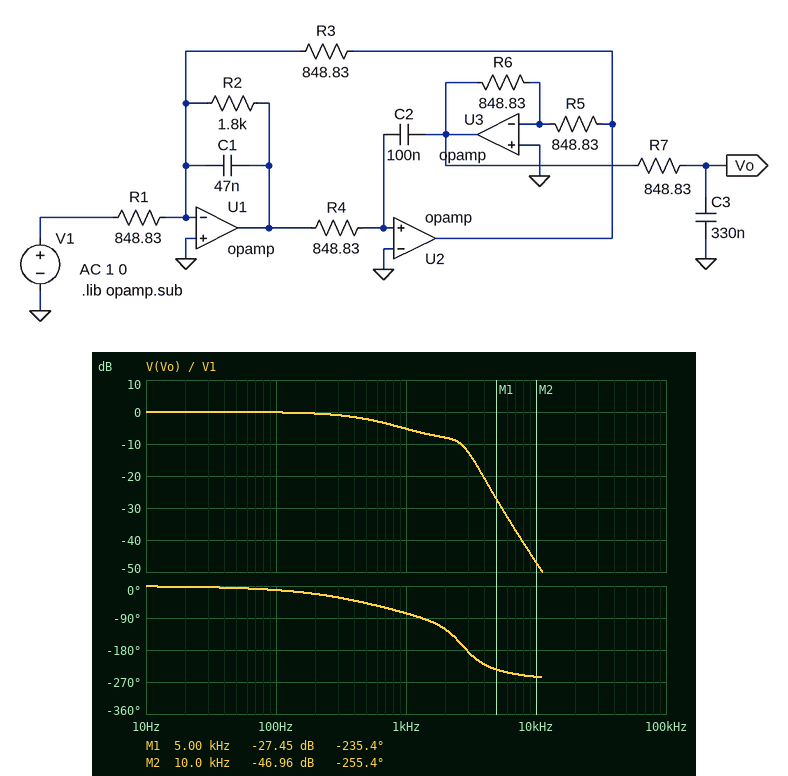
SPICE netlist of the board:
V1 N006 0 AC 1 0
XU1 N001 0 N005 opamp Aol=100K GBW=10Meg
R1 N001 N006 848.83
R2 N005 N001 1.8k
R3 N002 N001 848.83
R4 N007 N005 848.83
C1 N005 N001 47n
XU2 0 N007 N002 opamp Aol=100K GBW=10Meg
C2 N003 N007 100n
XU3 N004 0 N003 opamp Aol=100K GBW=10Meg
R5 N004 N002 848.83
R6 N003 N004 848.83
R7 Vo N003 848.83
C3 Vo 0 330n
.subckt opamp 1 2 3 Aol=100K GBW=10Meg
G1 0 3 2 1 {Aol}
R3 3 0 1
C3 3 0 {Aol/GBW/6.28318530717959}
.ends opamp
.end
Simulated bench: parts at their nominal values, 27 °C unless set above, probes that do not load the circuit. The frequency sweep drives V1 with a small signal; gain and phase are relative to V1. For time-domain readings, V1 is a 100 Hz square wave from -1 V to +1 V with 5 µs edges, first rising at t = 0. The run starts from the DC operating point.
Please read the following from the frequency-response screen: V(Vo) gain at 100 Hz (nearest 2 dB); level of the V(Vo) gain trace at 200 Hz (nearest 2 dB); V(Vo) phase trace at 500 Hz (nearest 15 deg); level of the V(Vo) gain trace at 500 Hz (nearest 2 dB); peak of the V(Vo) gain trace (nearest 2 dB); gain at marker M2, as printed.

0 dB
0 dB
-45 deg
-2 dB
0 dB
-46.96 dB
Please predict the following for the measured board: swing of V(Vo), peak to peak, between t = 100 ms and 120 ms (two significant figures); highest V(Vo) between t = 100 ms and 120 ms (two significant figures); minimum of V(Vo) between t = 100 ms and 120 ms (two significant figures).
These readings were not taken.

2.0 V
1.0 V
-1.0 V
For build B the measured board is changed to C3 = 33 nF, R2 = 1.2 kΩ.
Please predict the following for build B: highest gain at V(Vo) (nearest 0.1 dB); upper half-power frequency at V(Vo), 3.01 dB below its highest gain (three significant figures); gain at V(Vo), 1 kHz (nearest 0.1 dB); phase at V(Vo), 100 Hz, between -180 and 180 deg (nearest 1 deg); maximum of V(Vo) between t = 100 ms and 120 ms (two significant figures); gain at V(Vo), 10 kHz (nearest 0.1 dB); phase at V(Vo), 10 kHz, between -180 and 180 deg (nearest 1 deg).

0.7 dB
3.01 kHz
0.4 dB
-3 deg
1.3 V
-28.4 dB
136 deg
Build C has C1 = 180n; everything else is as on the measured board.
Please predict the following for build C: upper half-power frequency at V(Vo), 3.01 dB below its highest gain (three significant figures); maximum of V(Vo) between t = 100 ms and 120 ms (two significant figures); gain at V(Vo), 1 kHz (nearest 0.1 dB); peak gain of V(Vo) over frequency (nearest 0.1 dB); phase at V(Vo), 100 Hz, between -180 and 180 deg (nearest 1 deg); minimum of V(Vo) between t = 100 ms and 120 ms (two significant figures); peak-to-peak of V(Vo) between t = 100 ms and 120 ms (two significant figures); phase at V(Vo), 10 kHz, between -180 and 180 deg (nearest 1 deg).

1.53 kHz
1.1 V
-0.9 dB
1.1 dB
-11 deg
-1.1 V
2.2 V
96 deg
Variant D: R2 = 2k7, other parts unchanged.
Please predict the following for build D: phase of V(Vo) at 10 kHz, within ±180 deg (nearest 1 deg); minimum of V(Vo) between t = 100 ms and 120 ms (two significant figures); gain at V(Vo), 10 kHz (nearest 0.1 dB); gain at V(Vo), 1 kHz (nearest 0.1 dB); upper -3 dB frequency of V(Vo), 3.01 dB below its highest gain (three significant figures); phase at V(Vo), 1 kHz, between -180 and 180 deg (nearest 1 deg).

101 deg
-1.0 V
-46.9 dB
-5.0 dB
622 Hz
-71 deg
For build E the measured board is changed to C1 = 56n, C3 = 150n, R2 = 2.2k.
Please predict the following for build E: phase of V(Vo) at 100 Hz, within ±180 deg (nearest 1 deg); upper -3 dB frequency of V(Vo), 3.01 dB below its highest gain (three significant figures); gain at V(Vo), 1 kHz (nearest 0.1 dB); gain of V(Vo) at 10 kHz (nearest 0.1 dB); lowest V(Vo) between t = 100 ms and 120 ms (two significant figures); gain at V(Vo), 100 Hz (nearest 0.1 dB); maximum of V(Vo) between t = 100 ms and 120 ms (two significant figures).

-6 deg
2.72 kHz
-0.9 dB
-41.7 dB
-1.1 V
0 dB
1.1 V
